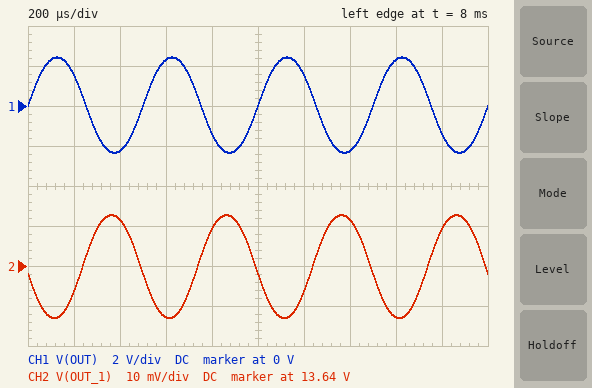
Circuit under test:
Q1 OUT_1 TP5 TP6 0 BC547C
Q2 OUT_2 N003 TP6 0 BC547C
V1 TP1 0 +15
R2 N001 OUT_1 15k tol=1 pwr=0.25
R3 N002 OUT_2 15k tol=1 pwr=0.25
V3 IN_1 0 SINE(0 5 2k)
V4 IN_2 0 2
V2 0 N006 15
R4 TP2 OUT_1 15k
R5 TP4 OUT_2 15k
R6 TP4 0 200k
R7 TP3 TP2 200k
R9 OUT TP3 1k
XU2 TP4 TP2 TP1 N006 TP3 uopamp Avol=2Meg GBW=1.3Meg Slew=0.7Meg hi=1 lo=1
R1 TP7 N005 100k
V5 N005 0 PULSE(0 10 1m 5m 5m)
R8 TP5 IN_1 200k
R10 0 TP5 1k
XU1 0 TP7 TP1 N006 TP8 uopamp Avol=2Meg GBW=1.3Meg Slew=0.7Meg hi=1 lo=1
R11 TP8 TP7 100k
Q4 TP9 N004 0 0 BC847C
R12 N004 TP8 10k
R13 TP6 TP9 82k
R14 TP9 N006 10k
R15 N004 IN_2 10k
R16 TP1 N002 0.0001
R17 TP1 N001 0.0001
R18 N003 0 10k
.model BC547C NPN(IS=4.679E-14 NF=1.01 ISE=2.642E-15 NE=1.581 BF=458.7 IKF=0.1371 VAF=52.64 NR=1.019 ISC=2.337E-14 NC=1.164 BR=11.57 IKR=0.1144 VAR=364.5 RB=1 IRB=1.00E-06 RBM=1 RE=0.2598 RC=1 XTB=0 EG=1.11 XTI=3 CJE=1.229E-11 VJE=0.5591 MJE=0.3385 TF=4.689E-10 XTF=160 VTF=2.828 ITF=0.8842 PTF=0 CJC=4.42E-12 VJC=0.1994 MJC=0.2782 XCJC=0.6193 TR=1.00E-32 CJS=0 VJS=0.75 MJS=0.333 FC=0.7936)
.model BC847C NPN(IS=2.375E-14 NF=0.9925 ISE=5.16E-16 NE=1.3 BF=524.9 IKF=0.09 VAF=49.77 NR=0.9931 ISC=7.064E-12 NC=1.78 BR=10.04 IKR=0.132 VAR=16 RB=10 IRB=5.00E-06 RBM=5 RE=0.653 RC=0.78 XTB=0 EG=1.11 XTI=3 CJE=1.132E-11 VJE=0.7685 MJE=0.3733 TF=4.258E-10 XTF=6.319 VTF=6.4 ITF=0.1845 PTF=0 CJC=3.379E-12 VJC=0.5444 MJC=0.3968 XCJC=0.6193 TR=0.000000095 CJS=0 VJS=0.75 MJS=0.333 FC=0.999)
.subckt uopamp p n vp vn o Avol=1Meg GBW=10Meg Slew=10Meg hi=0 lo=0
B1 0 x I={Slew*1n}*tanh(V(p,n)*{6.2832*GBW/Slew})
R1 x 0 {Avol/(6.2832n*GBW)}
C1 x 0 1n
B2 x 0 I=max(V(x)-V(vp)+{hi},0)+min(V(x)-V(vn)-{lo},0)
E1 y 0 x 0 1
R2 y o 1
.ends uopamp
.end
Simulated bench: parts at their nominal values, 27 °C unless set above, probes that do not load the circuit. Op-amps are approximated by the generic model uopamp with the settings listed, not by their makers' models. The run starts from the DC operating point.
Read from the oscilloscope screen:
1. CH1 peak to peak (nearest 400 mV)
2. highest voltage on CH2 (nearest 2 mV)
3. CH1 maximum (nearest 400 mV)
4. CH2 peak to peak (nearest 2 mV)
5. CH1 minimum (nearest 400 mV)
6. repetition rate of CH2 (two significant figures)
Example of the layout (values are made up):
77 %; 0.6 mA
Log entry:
4.8 V; 13.652 V; 2.4 V; 26 mV; -2.4 V; 2.0 kHz
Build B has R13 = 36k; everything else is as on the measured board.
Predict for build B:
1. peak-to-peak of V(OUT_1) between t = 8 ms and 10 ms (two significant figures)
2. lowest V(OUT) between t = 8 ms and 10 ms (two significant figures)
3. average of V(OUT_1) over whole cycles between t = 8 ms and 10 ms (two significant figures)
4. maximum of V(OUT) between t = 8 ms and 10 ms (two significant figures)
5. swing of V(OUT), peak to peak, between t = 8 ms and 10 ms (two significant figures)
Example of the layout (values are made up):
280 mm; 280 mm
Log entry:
57 mV; -5.1 V; 13 V; 5.5 V; 11 V
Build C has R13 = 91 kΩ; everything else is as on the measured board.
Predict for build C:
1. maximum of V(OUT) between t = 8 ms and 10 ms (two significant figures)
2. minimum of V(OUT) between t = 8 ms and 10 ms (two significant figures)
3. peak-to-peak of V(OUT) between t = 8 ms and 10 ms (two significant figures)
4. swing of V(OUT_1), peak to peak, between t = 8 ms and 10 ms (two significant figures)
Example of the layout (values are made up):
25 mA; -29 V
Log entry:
2.2 V; -2.1 V; 4.3 V; 23 mV
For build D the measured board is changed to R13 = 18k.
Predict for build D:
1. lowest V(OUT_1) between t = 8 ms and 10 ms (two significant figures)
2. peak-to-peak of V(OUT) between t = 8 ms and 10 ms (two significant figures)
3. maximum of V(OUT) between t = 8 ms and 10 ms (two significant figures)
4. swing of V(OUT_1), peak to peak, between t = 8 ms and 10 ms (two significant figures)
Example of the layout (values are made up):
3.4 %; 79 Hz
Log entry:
12 V; 20 V; 11 V; 110 mV
